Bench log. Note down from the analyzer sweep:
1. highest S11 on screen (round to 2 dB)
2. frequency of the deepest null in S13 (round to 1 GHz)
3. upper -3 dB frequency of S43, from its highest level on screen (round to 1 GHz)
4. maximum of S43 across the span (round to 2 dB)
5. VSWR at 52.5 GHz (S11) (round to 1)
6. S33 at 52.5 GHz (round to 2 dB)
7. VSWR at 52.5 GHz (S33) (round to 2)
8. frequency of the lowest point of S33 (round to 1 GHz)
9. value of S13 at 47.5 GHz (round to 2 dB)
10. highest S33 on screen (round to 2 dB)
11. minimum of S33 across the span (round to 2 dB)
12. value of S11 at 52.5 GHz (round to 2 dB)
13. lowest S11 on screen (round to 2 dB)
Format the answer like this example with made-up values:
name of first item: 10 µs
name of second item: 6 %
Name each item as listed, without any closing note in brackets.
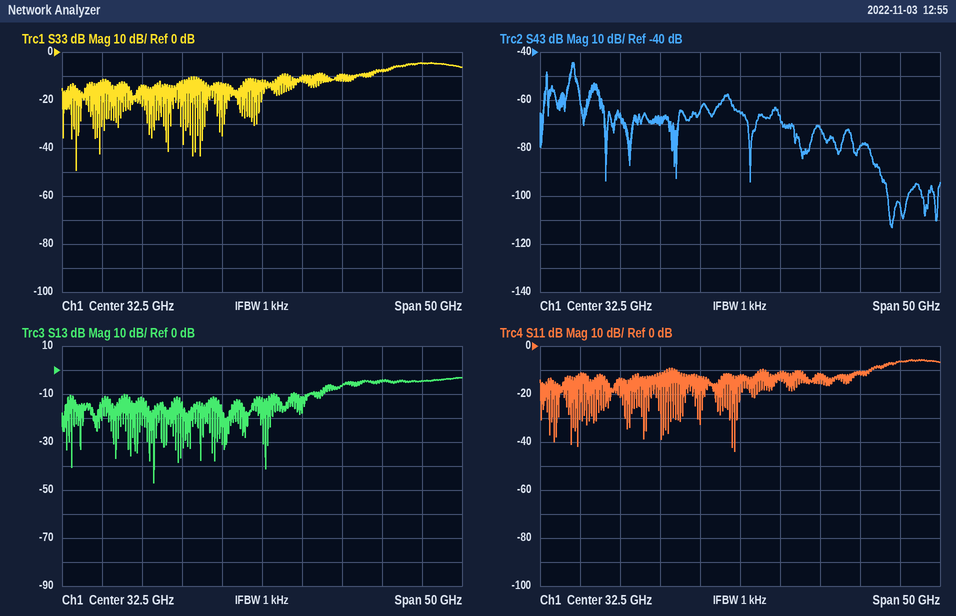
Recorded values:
highest S11 on screen: -6 dB
frequency of the deepest null in S13: 19 GHz
upper -3 dB frequency of S43, from its highest level on screen: 12 GHz
maximum of S43 across the span: -44 dB
VSWR at 52.5 GHz (S11): 3
S33 at 52.5 GHz: -4 dB
VSWR at 52.5 GHz (S33): 4
frequency of the lowest point of S33: 9 GHz
value of S13 at 47.5 GHz: -4 dB
highest S33 on screen: -4 dB
minimum of S33 across the span: -50 dB
value of S11 at 52.5 GHz: -6 dB
lowest S11 on screen: -44 dB
